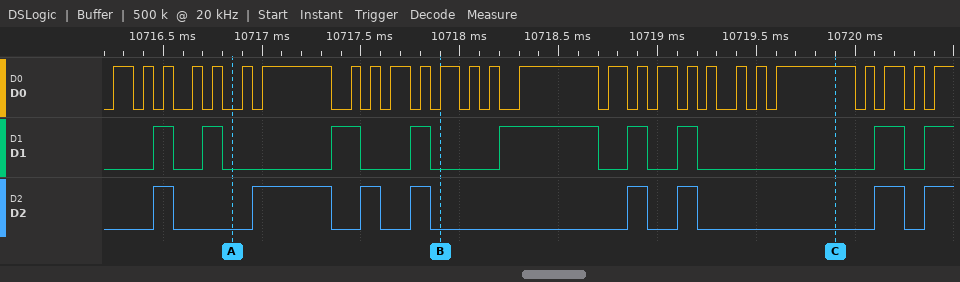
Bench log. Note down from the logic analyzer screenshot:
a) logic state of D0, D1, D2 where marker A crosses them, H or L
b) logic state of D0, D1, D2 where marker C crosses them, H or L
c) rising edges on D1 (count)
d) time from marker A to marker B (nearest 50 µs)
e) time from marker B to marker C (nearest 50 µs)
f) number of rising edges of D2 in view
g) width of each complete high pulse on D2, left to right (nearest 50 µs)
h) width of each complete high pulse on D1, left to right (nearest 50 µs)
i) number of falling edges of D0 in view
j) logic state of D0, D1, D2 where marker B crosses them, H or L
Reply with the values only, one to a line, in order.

D0=L, D1=L, D2=L
D0=H, D1=L, D2=L
9
1050 µs
2000 µs
8
100 µs, 400 µs, 100 µs, 100 µs, 100 µs, 100 µs, 150 µs
100 µs, 100 µs, 150 µs, 100 µs, 500 µs, 100 µs, 100 µs, 150 µs
26
D0=H, D1=L, D2=L
